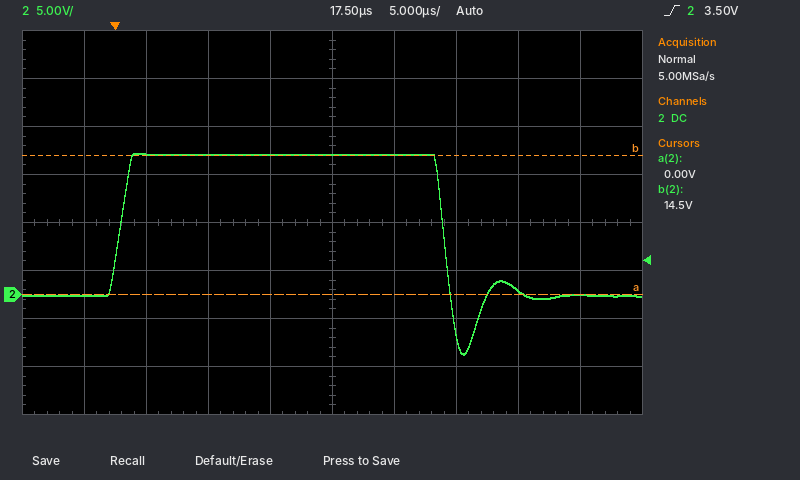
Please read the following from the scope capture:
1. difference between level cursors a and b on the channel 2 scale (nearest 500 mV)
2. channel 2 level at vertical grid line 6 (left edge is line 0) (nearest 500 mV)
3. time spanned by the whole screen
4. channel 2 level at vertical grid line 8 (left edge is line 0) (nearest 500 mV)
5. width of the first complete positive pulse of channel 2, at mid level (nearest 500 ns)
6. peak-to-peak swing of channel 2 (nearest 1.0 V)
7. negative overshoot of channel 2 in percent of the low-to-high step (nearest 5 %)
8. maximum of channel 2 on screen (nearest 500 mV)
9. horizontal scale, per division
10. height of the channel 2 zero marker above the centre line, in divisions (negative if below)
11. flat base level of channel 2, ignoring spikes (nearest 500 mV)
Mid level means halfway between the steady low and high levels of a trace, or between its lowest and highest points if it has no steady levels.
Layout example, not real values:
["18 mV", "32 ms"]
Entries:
["14.5 V", "14.5 V", "50 µs", "500 mV", "26.0 µs", "21.0 V", "40 %", "14.5 V", "5 µs", "-1.5 div", "0.0 V"]
